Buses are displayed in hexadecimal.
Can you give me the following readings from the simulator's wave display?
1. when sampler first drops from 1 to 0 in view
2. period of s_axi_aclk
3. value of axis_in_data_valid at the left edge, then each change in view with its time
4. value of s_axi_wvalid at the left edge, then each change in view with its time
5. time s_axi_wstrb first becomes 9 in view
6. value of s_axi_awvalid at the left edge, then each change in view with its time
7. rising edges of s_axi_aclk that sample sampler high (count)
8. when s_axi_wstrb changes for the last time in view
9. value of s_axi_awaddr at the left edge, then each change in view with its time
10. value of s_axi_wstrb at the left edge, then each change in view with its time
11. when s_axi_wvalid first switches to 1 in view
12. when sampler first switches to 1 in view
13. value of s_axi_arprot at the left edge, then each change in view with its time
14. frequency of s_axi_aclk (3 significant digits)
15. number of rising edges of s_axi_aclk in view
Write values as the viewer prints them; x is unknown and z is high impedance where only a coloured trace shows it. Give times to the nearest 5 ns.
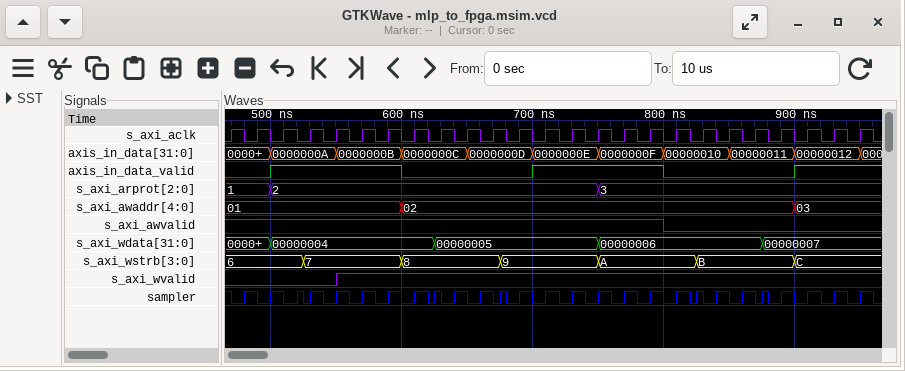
470 ns
20 ns
0, 1 at 500 ns, 0 at 600 ns, 1 at 700 ns, 0 at 800 ns, 1 at 900 ns
0, 1 at 550 ns
675 ns
1, 0 at 800 ns
9
900 ns
01, 02 at 600 ns, 03 at 900 ns
6, 7 at 525 ns, 8 at 600 ns, 9 at 675 ns, A at 750 ns, B at 825 ns, C at 900 ns
550 ns
480 ns
1, 2 at 500 ns, 3 at 750 ns
50.0 MHz
25
